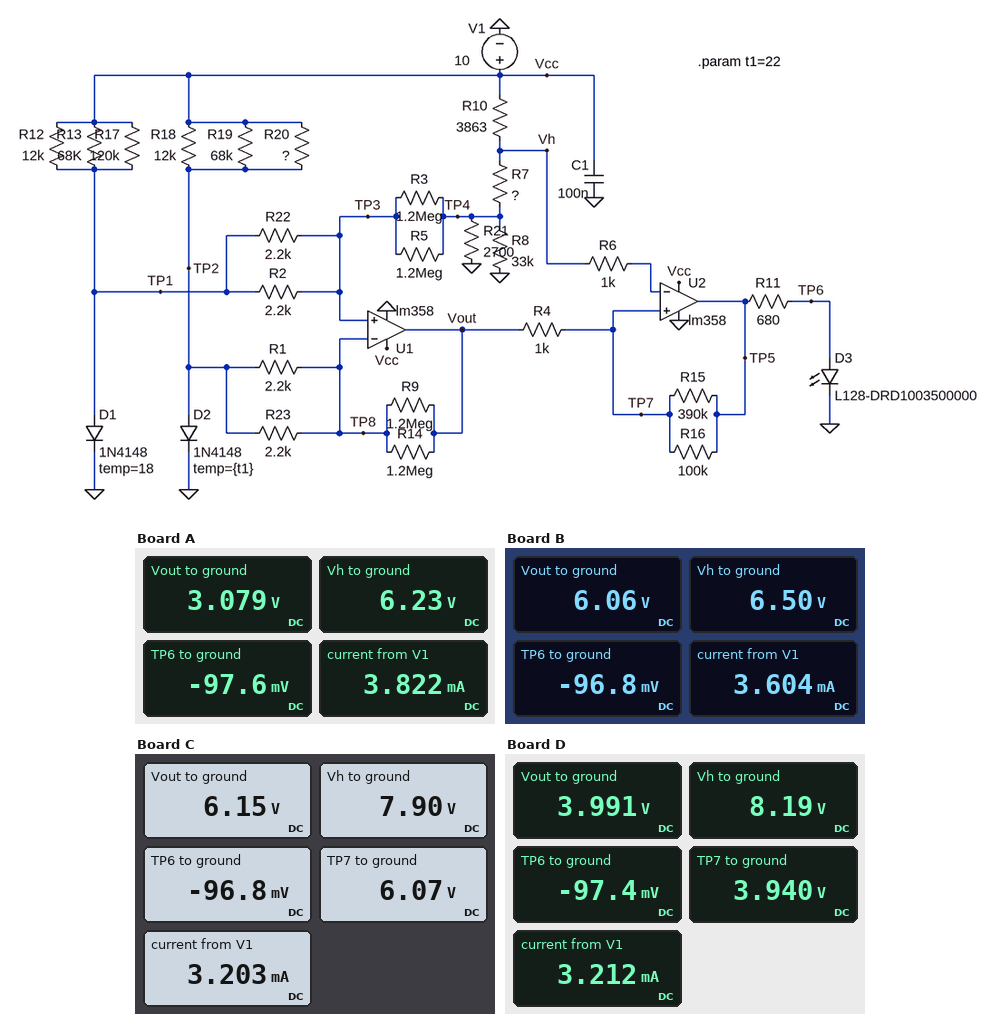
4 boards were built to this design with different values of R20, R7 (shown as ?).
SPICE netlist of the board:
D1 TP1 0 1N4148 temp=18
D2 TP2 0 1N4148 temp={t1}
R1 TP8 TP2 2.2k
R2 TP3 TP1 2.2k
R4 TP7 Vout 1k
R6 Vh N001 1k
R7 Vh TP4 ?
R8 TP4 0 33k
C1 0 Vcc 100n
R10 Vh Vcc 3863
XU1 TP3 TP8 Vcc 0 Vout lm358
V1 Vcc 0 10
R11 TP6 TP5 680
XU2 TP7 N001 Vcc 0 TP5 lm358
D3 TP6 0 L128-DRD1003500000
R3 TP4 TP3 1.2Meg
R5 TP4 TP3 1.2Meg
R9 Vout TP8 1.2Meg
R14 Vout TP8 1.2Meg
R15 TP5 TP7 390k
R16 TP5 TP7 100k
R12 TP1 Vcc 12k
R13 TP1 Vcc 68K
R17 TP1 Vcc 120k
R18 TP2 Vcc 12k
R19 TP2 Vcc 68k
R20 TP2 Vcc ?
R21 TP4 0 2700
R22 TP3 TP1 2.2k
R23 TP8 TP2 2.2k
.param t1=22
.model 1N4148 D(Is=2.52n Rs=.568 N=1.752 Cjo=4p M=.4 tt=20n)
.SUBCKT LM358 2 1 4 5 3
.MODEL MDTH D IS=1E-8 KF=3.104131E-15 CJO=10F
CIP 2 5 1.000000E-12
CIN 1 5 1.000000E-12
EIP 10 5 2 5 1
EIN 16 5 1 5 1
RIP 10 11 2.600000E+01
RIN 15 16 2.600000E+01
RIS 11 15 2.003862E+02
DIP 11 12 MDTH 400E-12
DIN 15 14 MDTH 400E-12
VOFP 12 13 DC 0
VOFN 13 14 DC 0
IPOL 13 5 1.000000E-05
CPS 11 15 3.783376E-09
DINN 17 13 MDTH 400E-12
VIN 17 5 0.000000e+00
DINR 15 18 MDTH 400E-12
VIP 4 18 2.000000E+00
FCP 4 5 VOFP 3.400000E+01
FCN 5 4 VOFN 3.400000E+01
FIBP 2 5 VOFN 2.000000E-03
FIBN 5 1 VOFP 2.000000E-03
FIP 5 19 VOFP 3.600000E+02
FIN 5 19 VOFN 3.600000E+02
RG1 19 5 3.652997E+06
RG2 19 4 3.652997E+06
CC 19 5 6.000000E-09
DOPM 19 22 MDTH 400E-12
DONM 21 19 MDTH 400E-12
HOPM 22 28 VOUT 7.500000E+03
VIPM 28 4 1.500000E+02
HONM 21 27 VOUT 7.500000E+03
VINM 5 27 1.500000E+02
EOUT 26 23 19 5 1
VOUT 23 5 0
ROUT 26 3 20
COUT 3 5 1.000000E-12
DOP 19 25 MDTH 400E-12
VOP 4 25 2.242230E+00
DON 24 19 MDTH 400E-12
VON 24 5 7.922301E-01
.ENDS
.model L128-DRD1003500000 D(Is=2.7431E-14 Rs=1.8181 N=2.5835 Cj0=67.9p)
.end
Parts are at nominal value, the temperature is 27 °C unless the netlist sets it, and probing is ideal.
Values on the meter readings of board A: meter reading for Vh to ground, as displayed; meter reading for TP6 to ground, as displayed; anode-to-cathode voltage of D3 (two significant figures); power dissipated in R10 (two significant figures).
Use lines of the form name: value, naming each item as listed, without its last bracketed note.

meter reading for Vh to ground, as displayed: 6.23 V
meter reading for TP6 to ground, as displayed: -97.6 mV
anode-to-cathode voltage of D3: -98 mV
power dissipated in R10: 3.7 mW
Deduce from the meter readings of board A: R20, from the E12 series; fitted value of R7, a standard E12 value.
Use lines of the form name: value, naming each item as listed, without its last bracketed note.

R20, from the E12 series: 39 kΩ
fitted value of R7, a standard E12 value: 3.9 kΩ
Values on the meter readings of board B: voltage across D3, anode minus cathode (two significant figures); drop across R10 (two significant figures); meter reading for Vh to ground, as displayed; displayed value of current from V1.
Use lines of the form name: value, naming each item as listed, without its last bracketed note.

voltage across D3, anode minus cathode: -97 mV
drop across R10: 3.5 V
meter reading for Vh to ground, as displayed: 6.50 V
displayed value of current from V1: 3.604 mA
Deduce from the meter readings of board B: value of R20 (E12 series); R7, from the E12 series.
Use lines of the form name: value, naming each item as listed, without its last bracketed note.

value of R20: 100 kΩ
R7, from the E12 series: 4.7 kΩ
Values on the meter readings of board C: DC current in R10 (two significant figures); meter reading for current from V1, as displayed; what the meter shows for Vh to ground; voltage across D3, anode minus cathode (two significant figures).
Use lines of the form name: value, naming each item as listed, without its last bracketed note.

DC current in R10: 540 µA
meter reading for current from V1, as displayed: 3.203 mA
what the meter shows for Vh to ground: 7.90 V
voltage across D3, anode minus cathode: -97 mV
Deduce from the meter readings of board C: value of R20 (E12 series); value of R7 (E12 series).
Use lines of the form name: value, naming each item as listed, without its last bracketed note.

value of R20: 180 kΩ
value of R7: 12 kΩ
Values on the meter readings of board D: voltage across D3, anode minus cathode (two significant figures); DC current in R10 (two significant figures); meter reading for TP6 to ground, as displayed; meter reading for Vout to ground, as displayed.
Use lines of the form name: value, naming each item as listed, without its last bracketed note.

voltage across D3, anode minus cathode: -97 mV
DC current in R10: 470 µA
meter reading for TP6 to ground, as displayed: -97.4 mV
meter reading for Vout to ground, as displayed: 3.991 V
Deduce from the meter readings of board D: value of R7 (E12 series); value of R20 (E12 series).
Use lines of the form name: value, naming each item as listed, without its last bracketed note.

value of R7: 15 kΩ
value of R20: 68 kΩ
